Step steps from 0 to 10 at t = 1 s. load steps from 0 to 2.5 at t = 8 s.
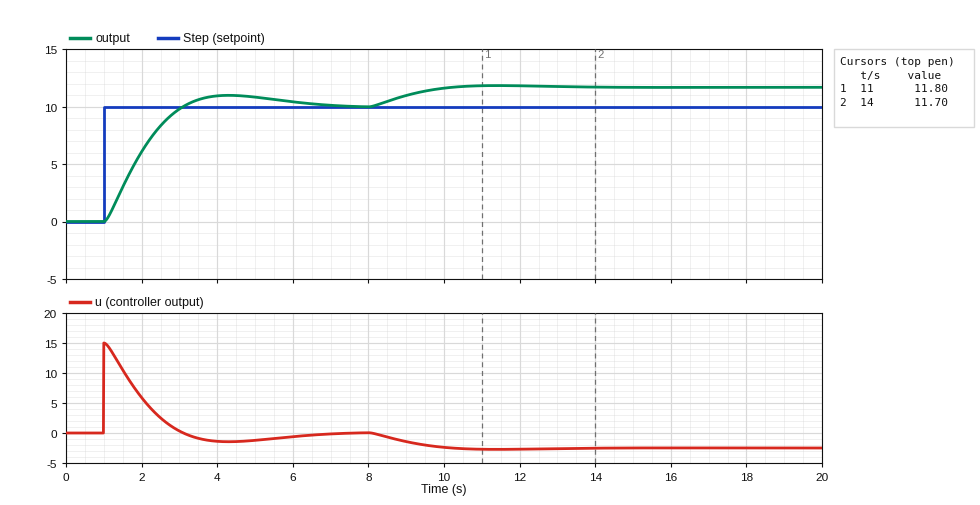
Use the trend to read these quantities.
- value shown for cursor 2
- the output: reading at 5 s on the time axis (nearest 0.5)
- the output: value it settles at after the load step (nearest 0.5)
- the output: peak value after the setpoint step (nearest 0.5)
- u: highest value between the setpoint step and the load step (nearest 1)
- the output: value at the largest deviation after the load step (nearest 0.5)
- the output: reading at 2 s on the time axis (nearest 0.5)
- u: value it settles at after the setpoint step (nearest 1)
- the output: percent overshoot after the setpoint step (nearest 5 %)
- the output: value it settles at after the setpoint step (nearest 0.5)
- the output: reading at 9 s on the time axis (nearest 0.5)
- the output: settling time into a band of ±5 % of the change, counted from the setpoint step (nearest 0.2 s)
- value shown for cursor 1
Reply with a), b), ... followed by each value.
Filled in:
a) 11.70
b) 11.0
c) 11.5
d) 11.0
e) 15
f) 12.0
g) 6.0
h) 0
i) 10 %
j) 10.0
k) 11.0
l) 4.8 s
m) 11.80
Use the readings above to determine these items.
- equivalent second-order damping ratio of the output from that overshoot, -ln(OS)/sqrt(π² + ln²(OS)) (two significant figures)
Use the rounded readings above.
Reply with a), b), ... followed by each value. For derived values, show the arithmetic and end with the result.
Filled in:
a) ln(0.1) = -2.303; 2.303 / sqrt(9.870 + 5.302) = 0.59
